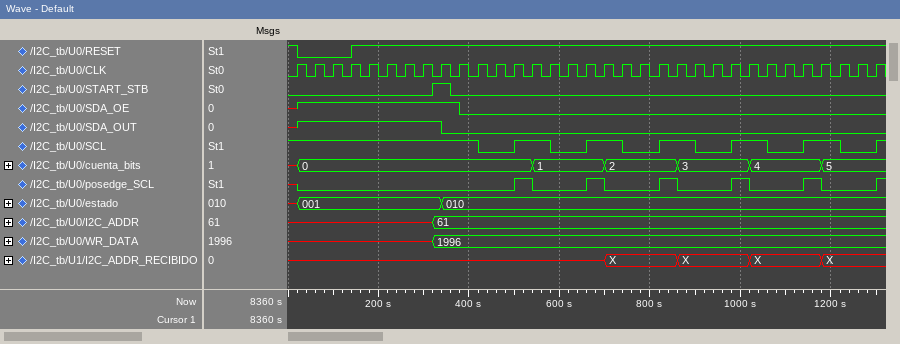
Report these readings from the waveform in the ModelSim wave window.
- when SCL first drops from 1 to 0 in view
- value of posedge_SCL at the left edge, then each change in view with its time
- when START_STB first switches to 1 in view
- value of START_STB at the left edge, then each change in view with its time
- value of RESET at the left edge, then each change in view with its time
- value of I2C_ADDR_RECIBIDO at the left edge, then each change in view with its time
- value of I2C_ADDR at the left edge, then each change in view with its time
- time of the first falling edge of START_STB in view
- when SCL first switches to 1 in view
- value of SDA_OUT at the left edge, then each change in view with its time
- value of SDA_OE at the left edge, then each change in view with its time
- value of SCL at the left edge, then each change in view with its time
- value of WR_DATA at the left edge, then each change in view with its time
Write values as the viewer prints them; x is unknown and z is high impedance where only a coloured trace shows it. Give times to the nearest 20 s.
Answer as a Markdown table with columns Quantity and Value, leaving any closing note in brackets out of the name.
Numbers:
| Quantity | Value |
|---|---|
| when SCL first drops from 1 to 0 in view | 420 s |
| value of posedge_SCL at the left edge, then each change in view with its time | x, 0 at 20 s, 1 at 500 s, 0 at 540 s, 1 at 660 s, 0 at 700 s, 1 at 820 s, 0 at 860 s, 1 at 980 s, 0 at 1020 s, 1 at 1140 s, 0 at 1180 s, 1 at 1300 s |
| when START_STB first switches to 1 in view | 320 s |
| value of START_STB at the left edge, then each change in view with its time | 0, 1 at 320 s, 0 at 360 s |
| value of RESET at the left edge, then each change in view with its time | 1, 0 at 20 s, 1 at 140 s |
| value of I2C_ADDR_RECIBIDO at the left edge, then each change in view with its time | x, X at 700 s, X at 860 s, X at 1020 s, X at 1180 s |
| value of I2C_ADDR at the left edge, then each change in view with its time | x, 61 at 320 s |
| time of the first falling edge of START_STB in view | 360 s |
| when SCL first switches to 1 in view | 500 s |
| value of SDA_OUT at the left edge, then each change in view with its time | x, 1 at 20 s, 0 at 340 s |
| value of SDA_OE at the left edge, then each change in view with its time | x, 1 at 20 s, 0 at 380 s |
| value of SCL at the left edge, then each change in view with its time | 1, 0 at 420 s, 1 at 500 s, 0 at 580 s, 1 at 660 s, 0 at 740 s, 1 at 820 s, 0 at 900 s, 1 at 980 s, 0 at 1060 s, 1 at 1140 s, 0 at 1220 s, 1 at 1300 s |
| value of WR_DATA at the left edge, then each change in view with its time | x, 1996 at 320 s |
